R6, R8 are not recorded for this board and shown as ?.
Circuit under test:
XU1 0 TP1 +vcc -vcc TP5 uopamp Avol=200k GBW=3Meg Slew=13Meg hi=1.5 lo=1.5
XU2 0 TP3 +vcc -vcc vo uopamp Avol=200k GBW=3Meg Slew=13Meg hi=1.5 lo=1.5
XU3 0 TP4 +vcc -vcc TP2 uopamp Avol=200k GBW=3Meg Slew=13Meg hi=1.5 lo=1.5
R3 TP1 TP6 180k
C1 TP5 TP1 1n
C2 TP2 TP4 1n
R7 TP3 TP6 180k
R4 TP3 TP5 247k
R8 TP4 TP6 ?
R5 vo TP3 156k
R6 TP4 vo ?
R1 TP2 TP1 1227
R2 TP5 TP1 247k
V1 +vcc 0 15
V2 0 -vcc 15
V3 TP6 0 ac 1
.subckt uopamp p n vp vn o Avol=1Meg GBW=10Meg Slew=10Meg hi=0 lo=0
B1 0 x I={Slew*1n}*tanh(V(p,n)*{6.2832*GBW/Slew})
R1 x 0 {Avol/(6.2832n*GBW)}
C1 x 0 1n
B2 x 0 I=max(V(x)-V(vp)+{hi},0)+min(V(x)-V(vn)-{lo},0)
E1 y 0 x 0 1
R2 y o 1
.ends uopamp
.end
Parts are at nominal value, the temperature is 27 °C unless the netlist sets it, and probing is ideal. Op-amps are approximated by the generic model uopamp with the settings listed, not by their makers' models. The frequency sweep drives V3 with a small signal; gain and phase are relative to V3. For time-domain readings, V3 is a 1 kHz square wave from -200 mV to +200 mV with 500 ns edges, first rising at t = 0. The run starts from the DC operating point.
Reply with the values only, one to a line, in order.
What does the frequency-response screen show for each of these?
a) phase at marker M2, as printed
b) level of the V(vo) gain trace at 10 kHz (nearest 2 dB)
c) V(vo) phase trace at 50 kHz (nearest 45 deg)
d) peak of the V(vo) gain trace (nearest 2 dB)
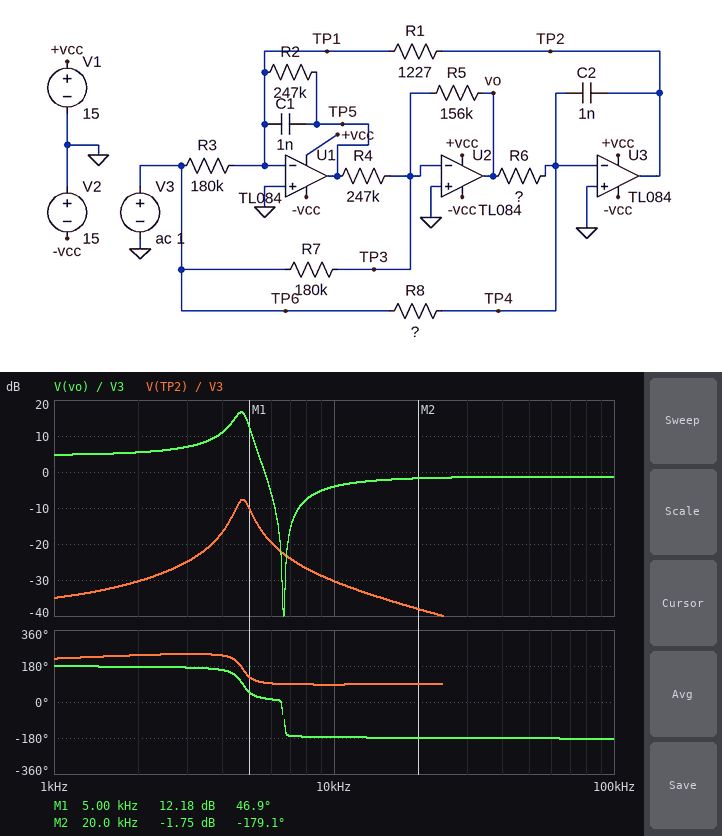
-179.1 deg
-4 dB
-180 deg
16 dB
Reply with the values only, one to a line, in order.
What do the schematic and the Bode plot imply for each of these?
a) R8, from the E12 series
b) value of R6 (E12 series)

330 kΩ
560 kΩ
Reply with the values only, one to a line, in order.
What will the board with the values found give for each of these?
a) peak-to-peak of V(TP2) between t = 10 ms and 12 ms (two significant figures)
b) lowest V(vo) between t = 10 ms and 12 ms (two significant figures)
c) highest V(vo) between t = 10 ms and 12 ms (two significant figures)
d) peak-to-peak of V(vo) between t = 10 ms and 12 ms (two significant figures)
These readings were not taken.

49 mV
-670 mV
670 mV
1.3 V
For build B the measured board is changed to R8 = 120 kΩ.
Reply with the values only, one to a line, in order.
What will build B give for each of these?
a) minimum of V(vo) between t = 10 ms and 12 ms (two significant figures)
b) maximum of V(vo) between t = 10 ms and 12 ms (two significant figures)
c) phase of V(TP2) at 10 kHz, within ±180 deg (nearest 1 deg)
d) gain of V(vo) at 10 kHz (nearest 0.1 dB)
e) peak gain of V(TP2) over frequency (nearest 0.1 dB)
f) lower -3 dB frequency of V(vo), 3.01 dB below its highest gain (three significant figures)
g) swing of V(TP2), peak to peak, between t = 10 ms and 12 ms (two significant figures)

-2.4 V
2.4 V
90 deg
-13.0 dB
5.4 dB
4.38 kHz
210 mV
